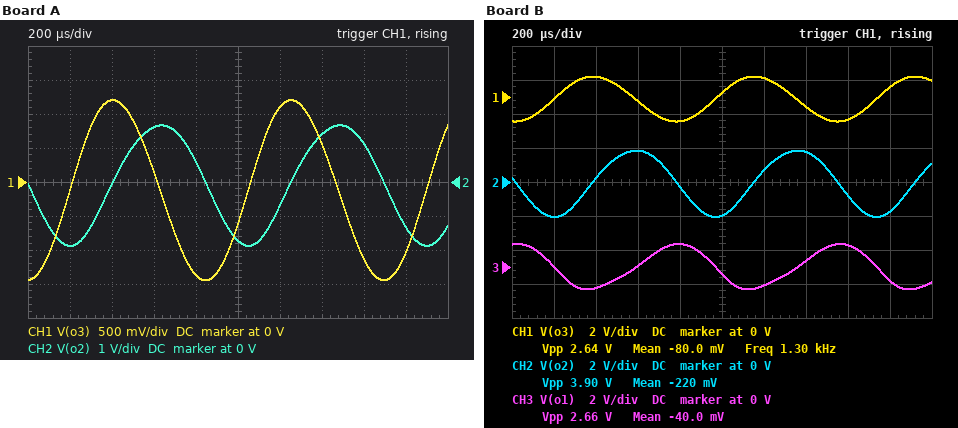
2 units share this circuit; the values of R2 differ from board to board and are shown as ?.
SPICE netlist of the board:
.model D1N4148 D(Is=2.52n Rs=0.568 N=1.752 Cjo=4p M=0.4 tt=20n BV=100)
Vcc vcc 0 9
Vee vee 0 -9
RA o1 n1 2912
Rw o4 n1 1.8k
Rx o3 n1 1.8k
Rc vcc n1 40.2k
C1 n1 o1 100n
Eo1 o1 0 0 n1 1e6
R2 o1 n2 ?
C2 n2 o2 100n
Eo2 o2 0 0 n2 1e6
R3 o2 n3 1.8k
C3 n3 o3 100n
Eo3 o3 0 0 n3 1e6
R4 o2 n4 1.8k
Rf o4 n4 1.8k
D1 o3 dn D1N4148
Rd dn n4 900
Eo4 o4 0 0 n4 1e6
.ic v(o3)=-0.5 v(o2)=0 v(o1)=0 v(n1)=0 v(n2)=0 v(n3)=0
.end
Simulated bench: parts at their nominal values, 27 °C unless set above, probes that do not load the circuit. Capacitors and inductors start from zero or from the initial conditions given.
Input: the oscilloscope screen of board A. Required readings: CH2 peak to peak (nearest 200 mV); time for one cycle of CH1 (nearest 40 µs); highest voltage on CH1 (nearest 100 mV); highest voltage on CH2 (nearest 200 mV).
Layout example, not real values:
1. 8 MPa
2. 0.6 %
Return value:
1. 3.6 V
2. 840 µs
3. 1.2 V
4. 1.6 V
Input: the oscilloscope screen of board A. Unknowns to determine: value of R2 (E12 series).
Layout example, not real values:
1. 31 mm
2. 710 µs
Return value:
1. 1 kΩ
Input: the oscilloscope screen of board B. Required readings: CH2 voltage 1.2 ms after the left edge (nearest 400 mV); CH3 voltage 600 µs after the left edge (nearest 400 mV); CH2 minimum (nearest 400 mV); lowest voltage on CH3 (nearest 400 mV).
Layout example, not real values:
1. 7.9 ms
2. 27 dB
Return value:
1. 800 mV
2. 0 V
3. -2.0 V
4. -1.2 V
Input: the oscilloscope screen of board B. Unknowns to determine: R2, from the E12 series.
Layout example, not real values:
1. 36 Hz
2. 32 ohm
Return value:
1. 820 Ω
